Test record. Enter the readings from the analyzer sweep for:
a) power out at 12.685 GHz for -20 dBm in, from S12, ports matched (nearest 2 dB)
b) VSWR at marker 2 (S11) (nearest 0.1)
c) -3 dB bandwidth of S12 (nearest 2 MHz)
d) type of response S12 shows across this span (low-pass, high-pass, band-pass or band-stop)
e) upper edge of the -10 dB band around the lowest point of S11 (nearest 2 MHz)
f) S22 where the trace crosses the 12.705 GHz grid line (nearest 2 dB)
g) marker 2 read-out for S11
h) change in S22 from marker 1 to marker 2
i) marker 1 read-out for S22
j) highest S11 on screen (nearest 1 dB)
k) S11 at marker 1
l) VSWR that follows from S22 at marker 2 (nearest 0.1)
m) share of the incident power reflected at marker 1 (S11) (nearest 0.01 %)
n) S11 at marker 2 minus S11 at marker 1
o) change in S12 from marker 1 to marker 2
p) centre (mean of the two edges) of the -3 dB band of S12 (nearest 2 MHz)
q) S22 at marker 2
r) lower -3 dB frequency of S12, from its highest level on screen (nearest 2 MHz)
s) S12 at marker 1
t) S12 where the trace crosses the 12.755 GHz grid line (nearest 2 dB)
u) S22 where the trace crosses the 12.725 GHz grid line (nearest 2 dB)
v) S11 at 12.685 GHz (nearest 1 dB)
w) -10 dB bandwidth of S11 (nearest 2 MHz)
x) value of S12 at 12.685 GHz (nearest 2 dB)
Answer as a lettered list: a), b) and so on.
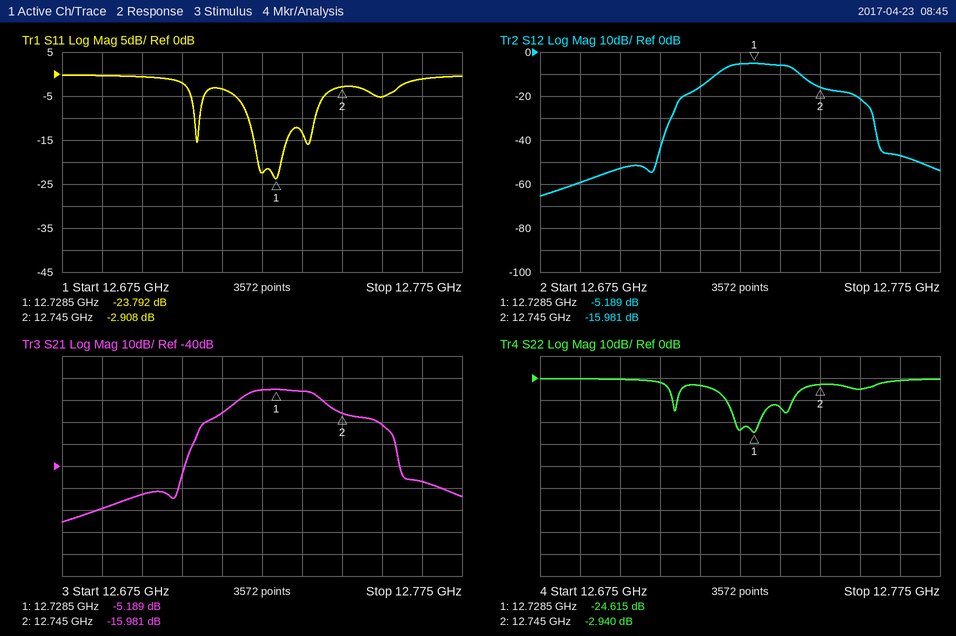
a) -80 dBm
b) 6.0
c) 18 MHz
d) band-pass
e) 12.738 GHz
f) -2 dB
g) -2.908 dB
h) 21.675 dB
i) -24.615 dB
j) 0 dB
k) -23.792 dB
l) 6.0
m) 0.42 %
n) 20.884 dB
o) -10.792 dB
p) 12.730 GHz
q) -2.940 dB
r) 12.720 GHz
s) -5.189 dB
t) -22 dB
u) -24 dB
v) 0 dB
w) 16 MHz
x) -60 dB
